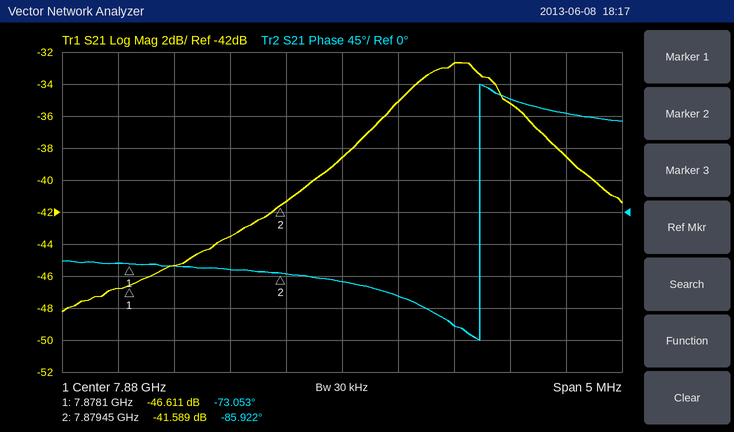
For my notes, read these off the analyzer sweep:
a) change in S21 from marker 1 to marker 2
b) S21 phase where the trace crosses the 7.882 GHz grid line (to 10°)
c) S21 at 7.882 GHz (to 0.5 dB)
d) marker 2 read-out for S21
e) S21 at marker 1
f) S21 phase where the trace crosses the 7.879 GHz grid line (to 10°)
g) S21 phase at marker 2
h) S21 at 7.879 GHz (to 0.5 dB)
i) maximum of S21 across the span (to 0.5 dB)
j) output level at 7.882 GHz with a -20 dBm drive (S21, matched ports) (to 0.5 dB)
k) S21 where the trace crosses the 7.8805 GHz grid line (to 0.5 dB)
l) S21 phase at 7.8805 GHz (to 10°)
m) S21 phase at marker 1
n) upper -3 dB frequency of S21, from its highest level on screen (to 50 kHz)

5.022 dB
140°
-38.5 dB
-41.589 dB
-46.611 dB
-80°
-85.922°
-43.5 dB
-32.5 dB
-58.5 dBm
-35.0 dB
-120°
-73.053°
7.88160 GHz
